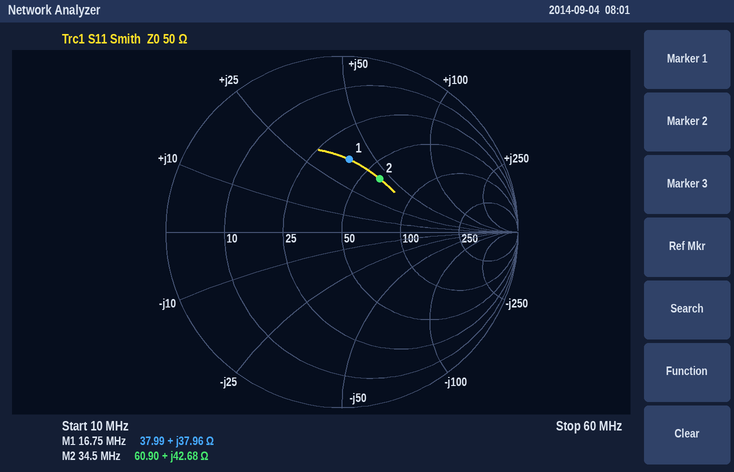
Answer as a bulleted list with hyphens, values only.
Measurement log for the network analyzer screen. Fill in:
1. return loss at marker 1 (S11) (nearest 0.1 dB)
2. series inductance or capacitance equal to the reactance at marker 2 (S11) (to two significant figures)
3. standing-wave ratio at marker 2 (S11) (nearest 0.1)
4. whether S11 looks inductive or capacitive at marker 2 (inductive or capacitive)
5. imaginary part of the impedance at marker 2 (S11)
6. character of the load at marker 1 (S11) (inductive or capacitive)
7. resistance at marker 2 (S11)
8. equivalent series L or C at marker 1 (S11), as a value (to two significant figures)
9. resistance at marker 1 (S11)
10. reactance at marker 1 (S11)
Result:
- 7.6 dB
- 200 nH
- 2.2
- inductive
- +42.68 Ω
- inductive
- 60.90 Ω
- 360 nH
- 37.99 Ω
- +37.96 Ω
